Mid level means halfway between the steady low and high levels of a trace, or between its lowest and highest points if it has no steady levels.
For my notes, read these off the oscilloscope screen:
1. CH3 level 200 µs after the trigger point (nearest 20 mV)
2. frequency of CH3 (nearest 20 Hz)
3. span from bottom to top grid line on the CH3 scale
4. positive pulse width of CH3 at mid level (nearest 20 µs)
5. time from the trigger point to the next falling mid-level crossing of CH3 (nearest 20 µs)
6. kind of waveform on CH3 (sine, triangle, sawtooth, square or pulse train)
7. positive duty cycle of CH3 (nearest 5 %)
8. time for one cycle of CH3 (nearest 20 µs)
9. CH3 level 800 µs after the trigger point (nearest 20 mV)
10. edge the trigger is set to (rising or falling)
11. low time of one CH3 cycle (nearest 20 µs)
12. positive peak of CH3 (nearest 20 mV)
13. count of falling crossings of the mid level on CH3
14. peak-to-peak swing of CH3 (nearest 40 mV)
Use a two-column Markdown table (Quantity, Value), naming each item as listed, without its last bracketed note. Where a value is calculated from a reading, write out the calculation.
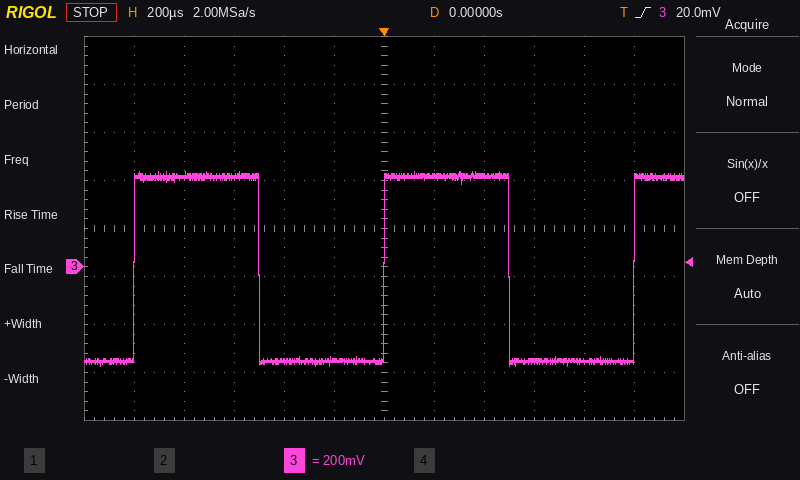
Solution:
| Quantity | Value |
|---|---|
| CH3 level 200 µs after the trigger point | 380 mV |
| frequency of CH3 | 1 / 1.00 ms ≈ 1.00 kHz |
| span from bottom to top grid line on the CH3 scale | 1.6 V |
| positive pulse width of CH3 at mid level | 500 µs |
| time from the trigger point to the next falling mid-level crossing of CH3 | 500 µs |
| kind of waveform on CH3 | square |
| positive duty cycle of CH3 | 500 µs / 1.00 ms ≈ 50 % |
| time for one cycle of CH3 | 1.00 ms |
| CH3 level 800 µs after the trigger point | -400 mV |
| edge the trigger is set to | rising |
| low time of one CH3 cycle | 500 µs |
| positive peak of CH3 | 400 mV |
| count of falling crossings of the mid level on CH3 | 2 |
| peak-to-peak swing of CH3 | 800 mV |
